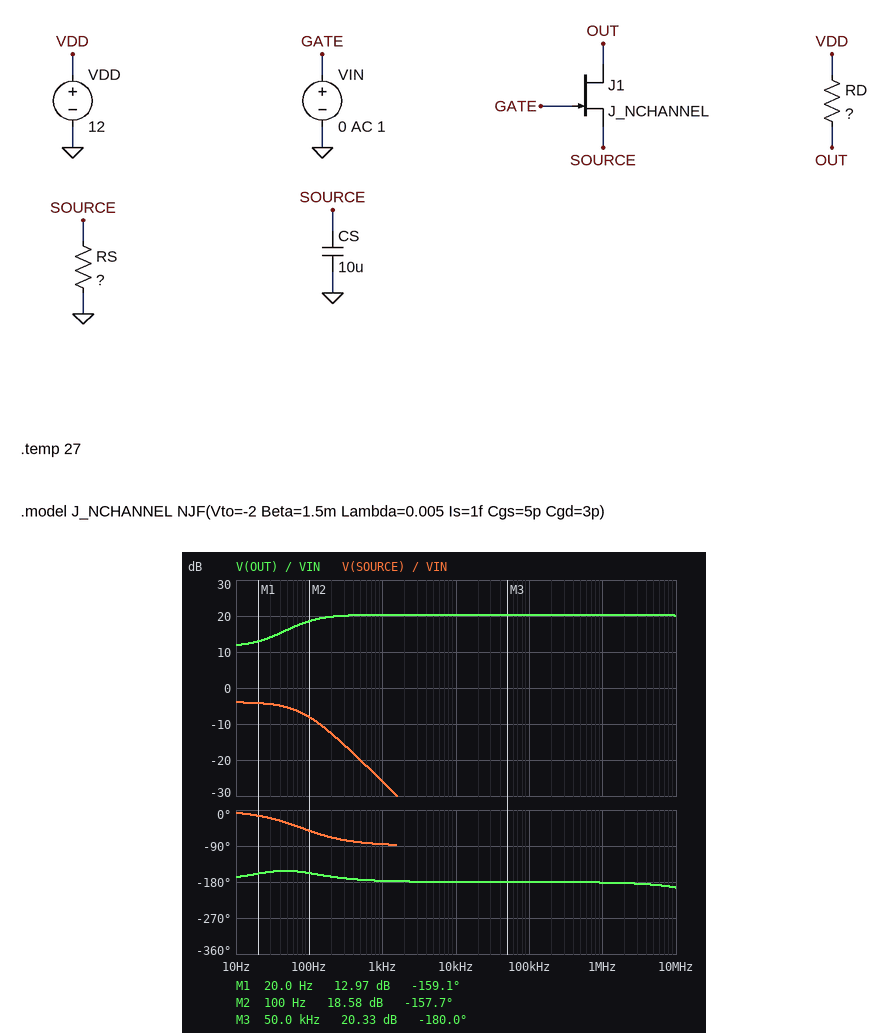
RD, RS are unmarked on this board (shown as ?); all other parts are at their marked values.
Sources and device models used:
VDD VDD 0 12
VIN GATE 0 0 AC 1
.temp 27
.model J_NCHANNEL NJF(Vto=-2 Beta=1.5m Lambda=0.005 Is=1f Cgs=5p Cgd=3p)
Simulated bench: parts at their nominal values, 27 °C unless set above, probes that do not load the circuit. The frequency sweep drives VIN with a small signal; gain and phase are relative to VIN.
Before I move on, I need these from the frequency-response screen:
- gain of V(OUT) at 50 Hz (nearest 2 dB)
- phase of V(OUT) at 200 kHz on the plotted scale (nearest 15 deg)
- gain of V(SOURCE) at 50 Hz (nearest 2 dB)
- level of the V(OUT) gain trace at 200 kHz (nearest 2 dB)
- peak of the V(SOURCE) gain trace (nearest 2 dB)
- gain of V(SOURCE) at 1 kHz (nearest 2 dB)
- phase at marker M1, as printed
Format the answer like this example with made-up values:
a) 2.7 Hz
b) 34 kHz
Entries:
a) 16 dB
b) -180 deg
c) -6 dB
d) 20 dB
e) -4 dB
f) -26 dB
g) -159.1 deg
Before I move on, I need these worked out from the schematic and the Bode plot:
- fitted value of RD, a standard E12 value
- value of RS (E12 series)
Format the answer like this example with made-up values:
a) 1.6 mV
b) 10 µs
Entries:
a) 3.3 kΩ
b) 560 Ω
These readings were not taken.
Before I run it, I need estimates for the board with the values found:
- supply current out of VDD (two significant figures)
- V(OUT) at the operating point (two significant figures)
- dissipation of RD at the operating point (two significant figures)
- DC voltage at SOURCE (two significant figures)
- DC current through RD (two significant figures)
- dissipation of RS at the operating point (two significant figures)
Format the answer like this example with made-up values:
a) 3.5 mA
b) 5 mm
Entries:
a) 1.7 mA
b) 6.4 V
c) 9.5 mW
d) 950 mV
e) 1.7 mA
f) 1.6 mW
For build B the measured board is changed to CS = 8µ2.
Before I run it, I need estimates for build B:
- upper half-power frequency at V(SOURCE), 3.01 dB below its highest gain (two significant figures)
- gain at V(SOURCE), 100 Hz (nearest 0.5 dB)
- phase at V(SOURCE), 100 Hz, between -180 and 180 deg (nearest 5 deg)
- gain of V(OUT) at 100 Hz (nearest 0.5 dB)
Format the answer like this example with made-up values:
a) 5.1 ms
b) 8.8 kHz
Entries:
a) 96 Hz
b) -7.0 dB
c) -45 deg
d) 18.0 dB
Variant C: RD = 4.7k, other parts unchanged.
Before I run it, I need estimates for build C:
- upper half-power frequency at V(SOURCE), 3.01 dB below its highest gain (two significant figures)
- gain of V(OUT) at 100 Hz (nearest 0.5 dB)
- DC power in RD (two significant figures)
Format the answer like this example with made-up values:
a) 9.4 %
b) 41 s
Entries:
a) 78 Hz
b) 21.5 dB
c) 13 mW
